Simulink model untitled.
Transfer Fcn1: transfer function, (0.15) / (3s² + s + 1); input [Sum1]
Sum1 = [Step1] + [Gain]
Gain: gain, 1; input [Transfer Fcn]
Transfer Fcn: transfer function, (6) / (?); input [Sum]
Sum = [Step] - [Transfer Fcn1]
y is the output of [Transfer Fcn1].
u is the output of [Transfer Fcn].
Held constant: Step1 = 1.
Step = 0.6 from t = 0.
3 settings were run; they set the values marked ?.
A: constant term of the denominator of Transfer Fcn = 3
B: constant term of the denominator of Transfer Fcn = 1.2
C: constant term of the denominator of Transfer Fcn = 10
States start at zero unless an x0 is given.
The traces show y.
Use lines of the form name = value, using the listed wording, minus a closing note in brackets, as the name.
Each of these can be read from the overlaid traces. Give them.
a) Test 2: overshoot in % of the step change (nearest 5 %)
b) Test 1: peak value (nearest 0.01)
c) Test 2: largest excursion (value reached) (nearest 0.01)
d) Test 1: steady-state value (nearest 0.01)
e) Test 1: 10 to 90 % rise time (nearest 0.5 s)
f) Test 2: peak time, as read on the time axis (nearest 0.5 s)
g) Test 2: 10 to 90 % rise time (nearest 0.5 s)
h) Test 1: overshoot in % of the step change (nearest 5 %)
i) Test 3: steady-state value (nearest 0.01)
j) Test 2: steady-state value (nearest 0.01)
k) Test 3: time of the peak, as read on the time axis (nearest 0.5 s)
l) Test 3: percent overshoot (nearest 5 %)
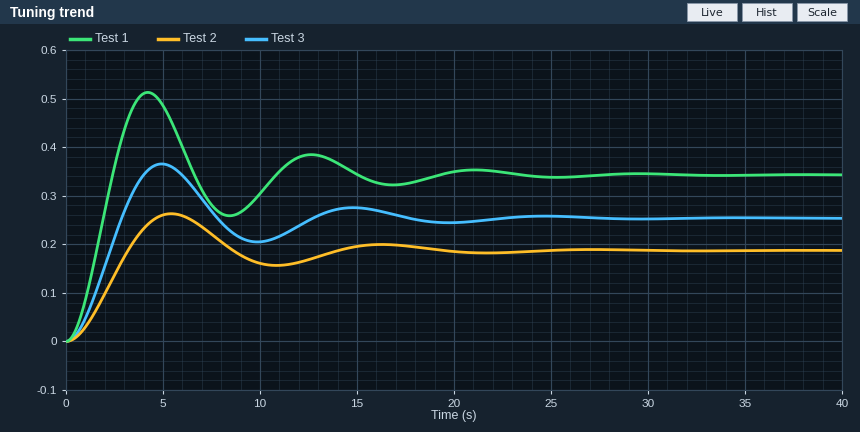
Test 2: overshoot in % of the step change = 40 %
Test 1: peak value = 0.51
Test 2: largest excursion (value reached) = 0.26
Test 1: steady-state value = 0.34
Test 1: 10 to 90 % rise time = 1.5 s
Test 2: peak time, as read on the time axis = 5.5 s
Test 2: 10 to 90 % rise time = 2.0 s
Test 1: overshoot in % of the step change = 50 %
Test 3: steady-state value = 0.25
Test 2: steady-state value = 0.19
Test 3: time of the peak, as read on the time axis = 5.0 s
Test 3: percent overshoot = 45 %
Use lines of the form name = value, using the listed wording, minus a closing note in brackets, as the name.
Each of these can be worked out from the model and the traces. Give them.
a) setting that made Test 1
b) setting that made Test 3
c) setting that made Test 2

setting that made Test 1 = B
setting that made Test 3 = A
setting that made Test 2 = C
